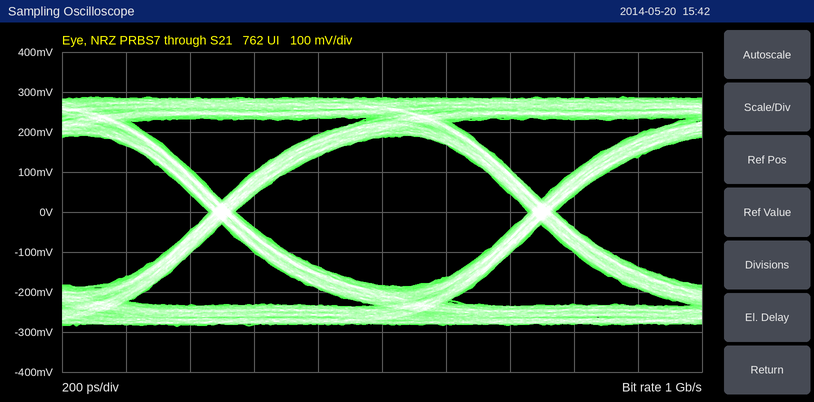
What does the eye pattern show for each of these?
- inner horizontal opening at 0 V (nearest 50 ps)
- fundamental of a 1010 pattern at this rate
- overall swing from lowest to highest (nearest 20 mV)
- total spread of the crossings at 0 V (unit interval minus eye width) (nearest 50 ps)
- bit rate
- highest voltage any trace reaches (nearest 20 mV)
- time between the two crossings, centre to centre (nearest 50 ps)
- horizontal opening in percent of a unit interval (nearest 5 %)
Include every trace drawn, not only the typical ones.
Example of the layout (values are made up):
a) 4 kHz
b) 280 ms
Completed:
a) 900 ps
b) 500 MHz
c) 580 mV
d) 100 ps
e) 1 Gb/s
f) 280 mV
g) 1.00 ns
h) 90 %
